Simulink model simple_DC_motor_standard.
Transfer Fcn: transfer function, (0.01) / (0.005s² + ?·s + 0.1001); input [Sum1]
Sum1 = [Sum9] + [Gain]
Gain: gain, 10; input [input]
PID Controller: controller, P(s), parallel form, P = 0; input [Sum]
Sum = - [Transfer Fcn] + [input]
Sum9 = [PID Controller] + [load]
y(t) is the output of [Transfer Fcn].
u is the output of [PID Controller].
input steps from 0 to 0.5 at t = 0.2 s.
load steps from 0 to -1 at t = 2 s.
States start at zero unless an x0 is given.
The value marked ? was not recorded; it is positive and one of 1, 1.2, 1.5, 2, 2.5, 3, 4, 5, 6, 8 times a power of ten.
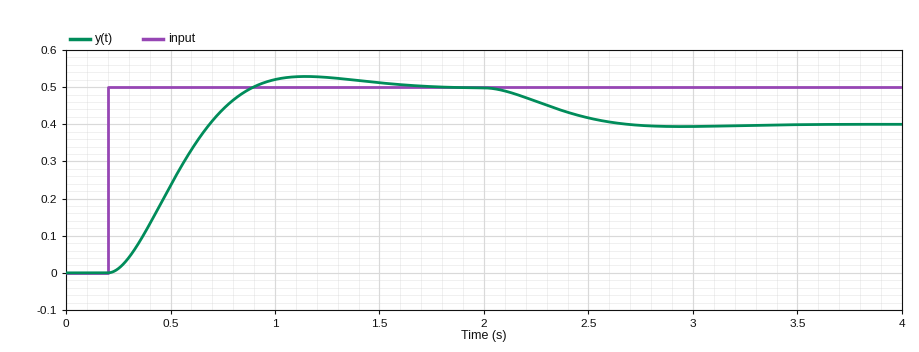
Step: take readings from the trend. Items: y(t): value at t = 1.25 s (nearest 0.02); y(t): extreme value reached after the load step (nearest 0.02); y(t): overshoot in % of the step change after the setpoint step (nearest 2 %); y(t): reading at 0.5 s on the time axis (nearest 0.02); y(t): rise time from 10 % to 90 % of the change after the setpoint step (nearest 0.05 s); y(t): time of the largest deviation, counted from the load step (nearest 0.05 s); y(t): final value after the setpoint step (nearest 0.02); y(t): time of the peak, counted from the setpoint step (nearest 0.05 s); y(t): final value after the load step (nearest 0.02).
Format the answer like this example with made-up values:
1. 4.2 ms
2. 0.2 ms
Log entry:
1. 0.52
2. 0.40
3. 6 %
4. 0.24
5. 0.45 s
6. 0.95 s
7. 0.50
8. 0.95 s
9. 0.40
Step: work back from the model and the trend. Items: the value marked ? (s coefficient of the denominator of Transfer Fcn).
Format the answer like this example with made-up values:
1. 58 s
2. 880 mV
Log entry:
1. 0.03
